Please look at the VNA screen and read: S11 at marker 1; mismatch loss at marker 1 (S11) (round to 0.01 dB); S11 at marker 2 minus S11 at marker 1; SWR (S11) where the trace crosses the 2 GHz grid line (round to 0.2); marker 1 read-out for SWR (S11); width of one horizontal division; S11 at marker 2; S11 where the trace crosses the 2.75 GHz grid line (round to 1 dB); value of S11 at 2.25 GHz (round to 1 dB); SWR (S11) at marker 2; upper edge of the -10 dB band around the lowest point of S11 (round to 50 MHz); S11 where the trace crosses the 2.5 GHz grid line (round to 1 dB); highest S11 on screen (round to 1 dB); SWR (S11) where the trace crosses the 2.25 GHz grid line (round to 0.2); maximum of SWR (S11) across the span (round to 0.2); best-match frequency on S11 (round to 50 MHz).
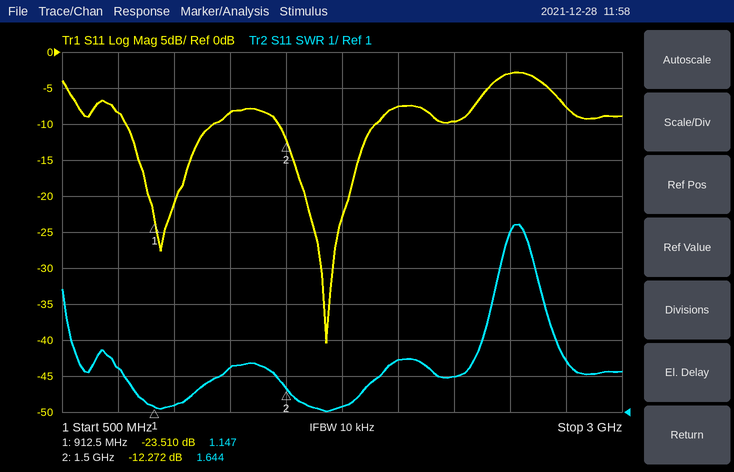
-23.510 dB
0.02 dB
11.238 dB
2.4
1.147
250 MHz
-12.272 dB
-8 dB
-10 dB
1.644
1.90 GHz
-3 dB
-3 dB
2.0
6.2
1.70 GHz
